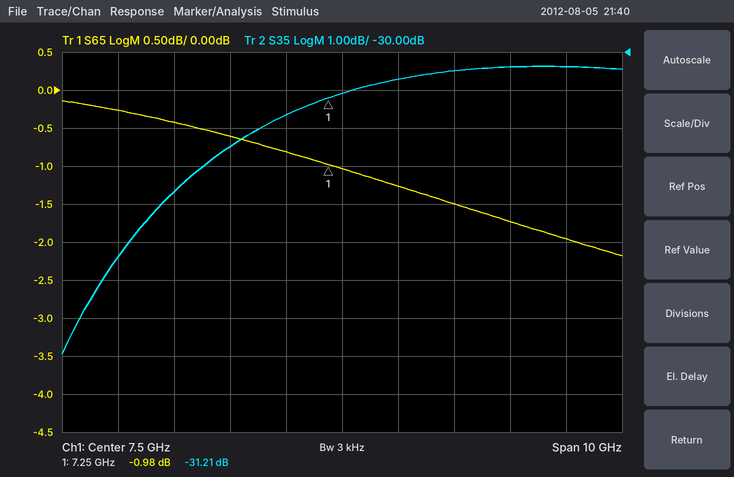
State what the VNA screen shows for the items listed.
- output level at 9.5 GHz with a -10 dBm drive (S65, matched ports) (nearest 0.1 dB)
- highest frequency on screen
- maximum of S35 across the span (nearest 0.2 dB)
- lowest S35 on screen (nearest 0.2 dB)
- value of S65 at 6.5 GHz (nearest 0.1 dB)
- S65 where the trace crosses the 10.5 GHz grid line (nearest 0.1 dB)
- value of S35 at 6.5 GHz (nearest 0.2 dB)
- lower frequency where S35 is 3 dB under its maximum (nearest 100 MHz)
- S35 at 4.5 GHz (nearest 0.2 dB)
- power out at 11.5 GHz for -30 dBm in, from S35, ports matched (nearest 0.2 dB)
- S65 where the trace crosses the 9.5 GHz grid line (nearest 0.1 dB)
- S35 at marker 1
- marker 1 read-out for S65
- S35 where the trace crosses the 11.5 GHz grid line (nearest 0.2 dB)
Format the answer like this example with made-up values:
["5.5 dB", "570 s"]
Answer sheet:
["-11.5 dBm", "12.5 GHz", "-30.4 dB", "-38.0 dB", "-0.8 dB", "-1.7 dB", "-31.6 dB", "4.7 GHz", "-33.6 dB", "-60.4 dBm", "-1.5 dB", "-31.21 dB", "-0.98 dB", "-30.4 dB"]
